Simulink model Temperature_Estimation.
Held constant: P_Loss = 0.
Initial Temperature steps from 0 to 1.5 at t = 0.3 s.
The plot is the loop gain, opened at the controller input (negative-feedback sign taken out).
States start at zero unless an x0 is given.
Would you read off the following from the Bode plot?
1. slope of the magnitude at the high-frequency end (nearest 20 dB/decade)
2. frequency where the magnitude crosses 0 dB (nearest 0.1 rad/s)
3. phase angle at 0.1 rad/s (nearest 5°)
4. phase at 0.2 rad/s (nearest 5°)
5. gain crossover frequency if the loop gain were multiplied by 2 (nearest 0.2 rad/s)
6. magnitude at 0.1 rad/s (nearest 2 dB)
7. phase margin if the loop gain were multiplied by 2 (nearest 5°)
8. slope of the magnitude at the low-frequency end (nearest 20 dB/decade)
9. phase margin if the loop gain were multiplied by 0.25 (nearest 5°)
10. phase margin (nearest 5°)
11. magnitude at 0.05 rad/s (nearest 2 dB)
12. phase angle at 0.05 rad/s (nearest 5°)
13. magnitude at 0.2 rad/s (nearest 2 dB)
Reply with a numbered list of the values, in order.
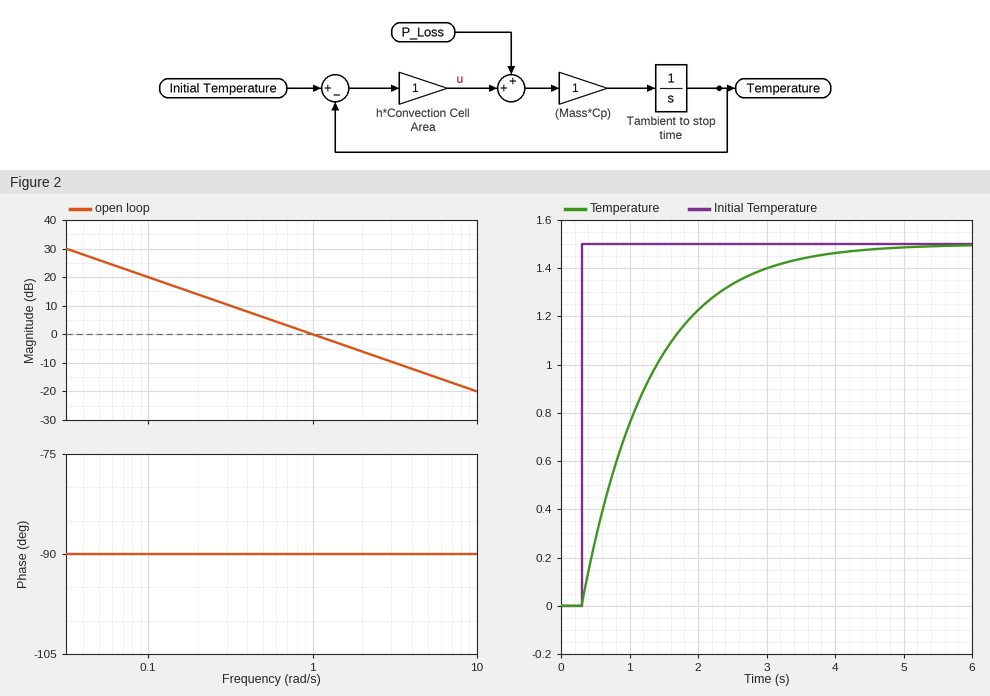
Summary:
1. -20 dB/decade
2. 1.0 rad/s
3. -90°
4. -90°
5. 2.0 rad/s
6. 20 dB
7. 90°
8. -20 dB/decade
9. 90°
10. 90°
11. 26 dB
12. -90°
13. 14 dB
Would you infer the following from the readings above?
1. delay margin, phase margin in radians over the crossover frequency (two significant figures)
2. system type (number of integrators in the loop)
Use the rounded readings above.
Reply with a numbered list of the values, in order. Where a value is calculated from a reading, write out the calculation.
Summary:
1. 90 × π / 180 / 1 = 1.6 s
2. 1
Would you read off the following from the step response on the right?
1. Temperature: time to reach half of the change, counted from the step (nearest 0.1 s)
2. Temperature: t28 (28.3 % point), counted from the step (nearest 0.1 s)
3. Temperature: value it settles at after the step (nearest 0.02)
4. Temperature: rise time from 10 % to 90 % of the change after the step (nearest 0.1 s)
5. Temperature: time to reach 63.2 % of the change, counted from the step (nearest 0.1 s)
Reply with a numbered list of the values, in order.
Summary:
1. 0.7 s
2. 0.3 s
3. 1.50
4. 2.2 s
5. 1.0 s
